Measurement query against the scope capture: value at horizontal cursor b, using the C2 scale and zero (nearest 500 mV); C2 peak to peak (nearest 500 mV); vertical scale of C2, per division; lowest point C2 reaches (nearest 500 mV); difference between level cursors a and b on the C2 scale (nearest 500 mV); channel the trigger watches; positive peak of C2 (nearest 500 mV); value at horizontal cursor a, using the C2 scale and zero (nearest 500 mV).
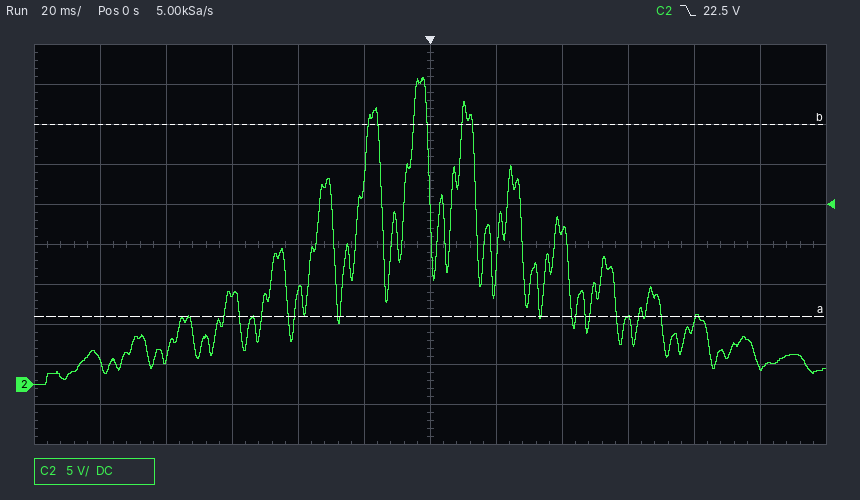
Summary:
32.5 V
38.5 V
5 V
0.0 V
24.0 V
C2
38.5 V
8.5 V
